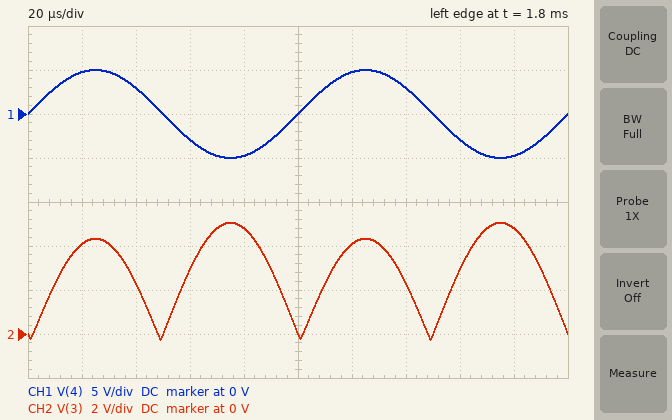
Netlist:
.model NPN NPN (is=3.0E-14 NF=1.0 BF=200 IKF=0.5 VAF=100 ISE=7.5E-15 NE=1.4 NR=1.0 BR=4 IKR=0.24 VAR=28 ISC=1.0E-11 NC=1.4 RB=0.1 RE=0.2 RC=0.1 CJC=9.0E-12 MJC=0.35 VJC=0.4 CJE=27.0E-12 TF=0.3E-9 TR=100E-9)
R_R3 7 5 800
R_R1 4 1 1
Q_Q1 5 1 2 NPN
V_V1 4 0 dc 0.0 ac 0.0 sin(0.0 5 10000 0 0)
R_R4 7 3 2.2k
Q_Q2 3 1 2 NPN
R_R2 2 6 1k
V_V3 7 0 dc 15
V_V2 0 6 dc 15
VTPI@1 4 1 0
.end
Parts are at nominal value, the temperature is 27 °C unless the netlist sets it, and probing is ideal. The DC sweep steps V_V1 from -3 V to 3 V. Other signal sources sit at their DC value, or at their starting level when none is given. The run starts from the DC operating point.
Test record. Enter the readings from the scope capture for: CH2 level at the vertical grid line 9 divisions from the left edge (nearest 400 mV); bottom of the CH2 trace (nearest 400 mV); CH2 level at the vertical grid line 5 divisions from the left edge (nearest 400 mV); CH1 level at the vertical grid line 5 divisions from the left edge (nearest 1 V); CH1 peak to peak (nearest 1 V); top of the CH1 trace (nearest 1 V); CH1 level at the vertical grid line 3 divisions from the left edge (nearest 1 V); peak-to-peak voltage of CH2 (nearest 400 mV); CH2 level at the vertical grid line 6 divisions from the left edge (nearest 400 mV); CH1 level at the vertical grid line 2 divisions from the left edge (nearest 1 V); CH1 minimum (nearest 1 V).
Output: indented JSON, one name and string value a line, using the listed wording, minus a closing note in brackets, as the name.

{
  "CH2 level at the vertical grid line 9 divisions from the left edge": "4.8 V",
  "bottom of the CH2 trace": "-400 mV",
  "CH2 level at the vertical grid line 5 divisions from the left edge": "0 V",
  "CH1 level at the vertical grid line 5 divisions from the left edge": "0 V",
  "CH1 peak to peak": "10 V",
  "top of the CH1 trace": "5 V",
  "CH1 level at the vertical grid line 3 divisions from the left edge": "-3 V",
  "peak-to-peak voltage of CH2": "5.2 V",
  "CH2 level at the vertical grid line 6 divisions from the left edge": "4.0 V",
  "CH1 level at the vertical grid line 2 divisions from the left edge": "3 V",
  "CH1 minimum": "-5 V"
}
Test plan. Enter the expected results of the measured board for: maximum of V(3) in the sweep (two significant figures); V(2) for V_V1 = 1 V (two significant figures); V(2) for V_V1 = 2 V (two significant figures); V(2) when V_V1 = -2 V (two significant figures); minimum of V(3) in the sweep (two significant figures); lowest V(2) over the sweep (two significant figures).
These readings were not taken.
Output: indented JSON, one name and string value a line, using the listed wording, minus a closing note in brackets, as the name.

{
  "maximum of V(3) in the sweep": "3.0 V",
  "V(2) for V_V1 = 1 V": "320 mV",
  "V(2) for V_V1 = 2 V": "1.3 V",
  "V(2) when V_V1 = -2 V": "-2.7 V",
  "minimum of V(3) in the sweep": "-240 mV",
  "lowest V(2) over the sweep": "-3.7 V"
}
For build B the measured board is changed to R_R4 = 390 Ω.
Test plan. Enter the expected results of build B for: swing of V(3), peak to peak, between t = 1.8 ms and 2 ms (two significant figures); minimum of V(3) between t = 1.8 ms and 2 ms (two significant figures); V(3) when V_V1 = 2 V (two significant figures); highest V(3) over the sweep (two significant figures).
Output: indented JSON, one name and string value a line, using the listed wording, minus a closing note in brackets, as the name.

{
  "swing of V(3), peak to peak, between t = 1.8 ms and 2 ms": "2.0 V",
  "minimum of V(3) between t = 1.8 ms and 2 ms": "11 V",
  "V(3) when V_V1 = 2 V": "12 V",
  "highest V(3) over the sweep": "13 V"
}
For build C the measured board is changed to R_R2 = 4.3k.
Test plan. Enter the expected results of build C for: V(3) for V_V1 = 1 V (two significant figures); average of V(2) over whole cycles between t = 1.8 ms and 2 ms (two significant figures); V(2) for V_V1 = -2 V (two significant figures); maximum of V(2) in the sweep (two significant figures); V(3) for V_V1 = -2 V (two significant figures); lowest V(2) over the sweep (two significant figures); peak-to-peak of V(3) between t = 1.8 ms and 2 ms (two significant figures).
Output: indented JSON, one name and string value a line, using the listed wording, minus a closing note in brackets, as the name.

{
  "V(3) for V_V1 = 1 V": "11 V",
  "average of V(2) over whole cycles between t = 1.8 ms and 2 ms": "-640 mV",
  "V(2) for V_V1 = -2 V": "-2.6 V",
  "maximum of V(2) in the sweep": "2.4 V",
  "V(3) for V_V1 = -2 V": "12 V",
  "lowest V(2) over the sweep": "-3.6 V",
  "peak-to-peak of V(3) between t = 1.8 ms and 2 ms": "2.5 V"
}
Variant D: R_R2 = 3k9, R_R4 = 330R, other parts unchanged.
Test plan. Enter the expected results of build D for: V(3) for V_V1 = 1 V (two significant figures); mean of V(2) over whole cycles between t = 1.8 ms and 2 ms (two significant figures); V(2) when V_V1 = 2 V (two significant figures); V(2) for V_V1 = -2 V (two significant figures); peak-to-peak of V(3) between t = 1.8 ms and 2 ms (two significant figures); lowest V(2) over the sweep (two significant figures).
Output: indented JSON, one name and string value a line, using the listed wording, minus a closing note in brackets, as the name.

{
  "V(3) for V_V1 = 1 V": "14 V",
  "mean of V(2) over whole cycles between t = 1.8 ms and 2 ms": "-640 mV",
  "V(2) when V_V1 = 2 V": "1.4 V",
  "V(2) for V_V1 = -2 V": "-2.6 V",
  "peak-to-peak of V(3) between t = 1.8 ms and 2 ms": "420 mV",
  "lowest V(2) over the sweep": "-3.6 V"
}
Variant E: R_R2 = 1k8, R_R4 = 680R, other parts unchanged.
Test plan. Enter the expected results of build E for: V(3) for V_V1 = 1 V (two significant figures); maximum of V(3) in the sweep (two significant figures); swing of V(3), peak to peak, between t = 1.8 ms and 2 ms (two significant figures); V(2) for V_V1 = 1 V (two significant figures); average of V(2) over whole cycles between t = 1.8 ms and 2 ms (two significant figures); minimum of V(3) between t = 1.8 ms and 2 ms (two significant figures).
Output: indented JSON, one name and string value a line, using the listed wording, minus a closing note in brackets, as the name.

{
  "V(3) for V_V1 = 1 V": "12 V",
  "maximum of V(3) in the sweep": "13 V",
  "swing of V(3), peak to peak, between t = 1.8 ms and 2 ms": "1.9 V",
  "V(2) for V_V1 = 1 V": "340 mV",
  "average of V(2) over whole cycles between t = 1.8 ms and 2 ms": "-660 mV",
  "minimum of V(3) between t = 1.8 ms and 2 ms": "11 V"
}
